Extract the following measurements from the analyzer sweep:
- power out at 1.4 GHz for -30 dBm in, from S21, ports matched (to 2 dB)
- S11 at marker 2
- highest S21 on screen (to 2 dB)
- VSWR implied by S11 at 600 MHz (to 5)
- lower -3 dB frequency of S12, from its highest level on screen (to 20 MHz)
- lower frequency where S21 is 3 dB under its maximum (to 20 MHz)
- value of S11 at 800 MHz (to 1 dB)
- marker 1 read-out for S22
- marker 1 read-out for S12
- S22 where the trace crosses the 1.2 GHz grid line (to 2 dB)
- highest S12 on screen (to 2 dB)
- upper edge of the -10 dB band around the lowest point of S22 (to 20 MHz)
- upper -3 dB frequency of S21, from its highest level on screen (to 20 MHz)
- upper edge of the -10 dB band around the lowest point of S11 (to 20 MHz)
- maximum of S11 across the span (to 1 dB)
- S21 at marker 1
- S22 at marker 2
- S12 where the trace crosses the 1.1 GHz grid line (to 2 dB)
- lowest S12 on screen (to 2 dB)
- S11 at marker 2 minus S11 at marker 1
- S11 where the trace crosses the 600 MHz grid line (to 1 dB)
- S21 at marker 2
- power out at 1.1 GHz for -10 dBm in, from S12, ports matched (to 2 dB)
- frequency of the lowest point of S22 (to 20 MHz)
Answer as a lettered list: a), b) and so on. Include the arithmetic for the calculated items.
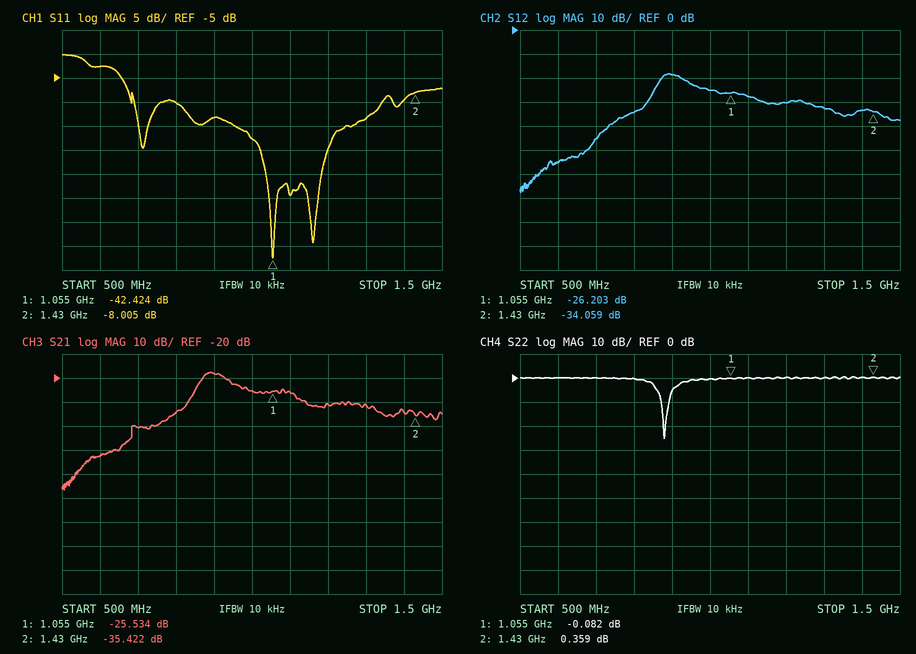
a) -30 dBm + (-34 dB) = -64 dBm
b) -8.005 dB
c) -18 dB
d) |Γ| = 10^(-3/20) = 0.7079; VSWR = (1 + 0.7079)/(1 − 0.7079) ≈ 5.85, so 5 to the nearest 5
e) 860 MHz
f) 860 MHz
g) -10 dB
h) -0.082 dB
i) -26.203 dB
j) 0 dB
k) -18 dB
l) 900 MHz
m) 940 MHz
n) 1.34 GHz
o) 0 dB
p) -25.534 dB
q) 0.359 dB
r) -28 dB
s) -68 dB
t) -8.005 − (-42.424) = 34.419 dB
u) -3 dB
v) -35.422 dB
w) -10 dBm + (-28 dB) = -38 dBm
x) 880 MHz
